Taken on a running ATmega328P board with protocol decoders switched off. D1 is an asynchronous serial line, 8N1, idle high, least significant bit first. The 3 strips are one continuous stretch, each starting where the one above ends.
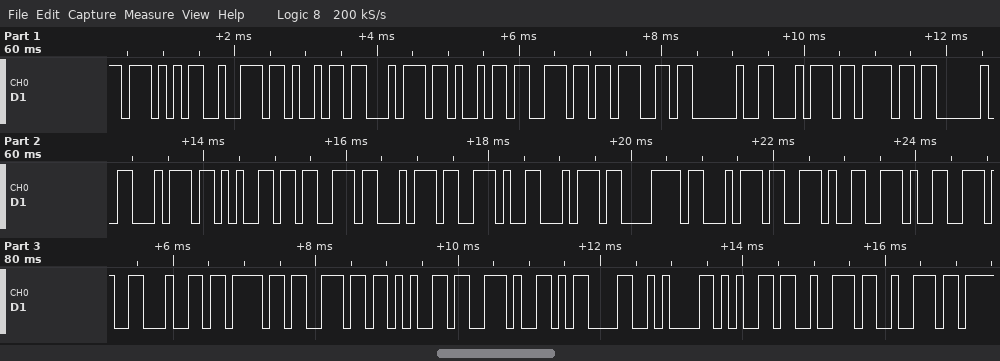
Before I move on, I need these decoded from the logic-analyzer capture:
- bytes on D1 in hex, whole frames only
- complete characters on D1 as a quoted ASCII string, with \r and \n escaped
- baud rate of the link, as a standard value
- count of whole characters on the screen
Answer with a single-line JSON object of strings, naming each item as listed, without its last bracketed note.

{"bytes on D1 in hex, whole frames only": "57 72 69 74 69 6E 67 20 74 6F 20 74 65 73 74 2E 74 78 74 2E 2E 2E 64 6F 6E 65 2E 0D 0A 65 72 72", "complete characters on D1 as a quoted ASCII string, with \\r and \\n escaped": "\"Writing to test.txt...done.\\r\\nerr\"", "baud rate of the link, as a standard value": "9600 baud", "count of whole characters on the screen": "32"}
